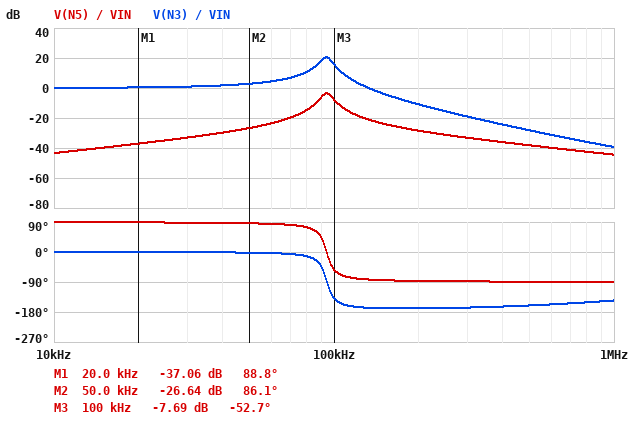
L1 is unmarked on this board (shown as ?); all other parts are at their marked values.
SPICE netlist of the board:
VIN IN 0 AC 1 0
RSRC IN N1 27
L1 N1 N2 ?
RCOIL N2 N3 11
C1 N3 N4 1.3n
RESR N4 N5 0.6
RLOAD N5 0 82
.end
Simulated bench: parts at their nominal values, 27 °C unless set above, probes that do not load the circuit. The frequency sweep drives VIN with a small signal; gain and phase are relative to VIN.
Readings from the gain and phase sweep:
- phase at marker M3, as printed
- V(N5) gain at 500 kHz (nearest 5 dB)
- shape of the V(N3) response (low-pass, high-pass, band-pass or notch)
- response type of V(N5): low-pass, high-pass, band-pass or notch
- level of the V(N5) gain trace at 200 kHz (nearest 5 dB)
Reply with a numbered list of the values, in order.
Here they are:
1. -52.7 deg
2. -40 dB
3. low-pass
4. band-pass
5. -30 dB
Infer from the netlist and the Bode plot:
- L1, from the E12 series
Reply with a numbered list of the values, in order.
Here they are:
1. 2.2 mH
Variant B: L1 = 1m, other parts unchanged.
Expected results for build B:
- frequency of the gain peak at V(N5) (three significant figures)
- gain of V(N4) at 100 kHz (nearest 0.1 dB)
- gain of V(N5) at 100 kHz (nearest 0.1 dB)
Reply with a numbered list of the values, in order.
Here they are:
1. 140 kHz
2. -17.3 dB
3. -17.4 dB
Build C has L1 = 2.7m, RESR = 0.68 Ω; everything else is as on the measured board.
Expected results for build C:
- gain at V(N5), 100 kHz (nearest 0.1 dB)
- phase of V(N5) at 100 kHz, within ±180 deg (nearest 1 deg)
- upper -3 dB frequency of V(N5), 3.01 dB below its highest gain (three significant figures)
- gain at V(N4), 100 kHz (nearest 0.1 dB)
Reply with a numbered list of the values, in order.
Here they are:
1. -15.5 dB
2. -76 deg
3. 88.6 kHz
4. -15.4 dB
